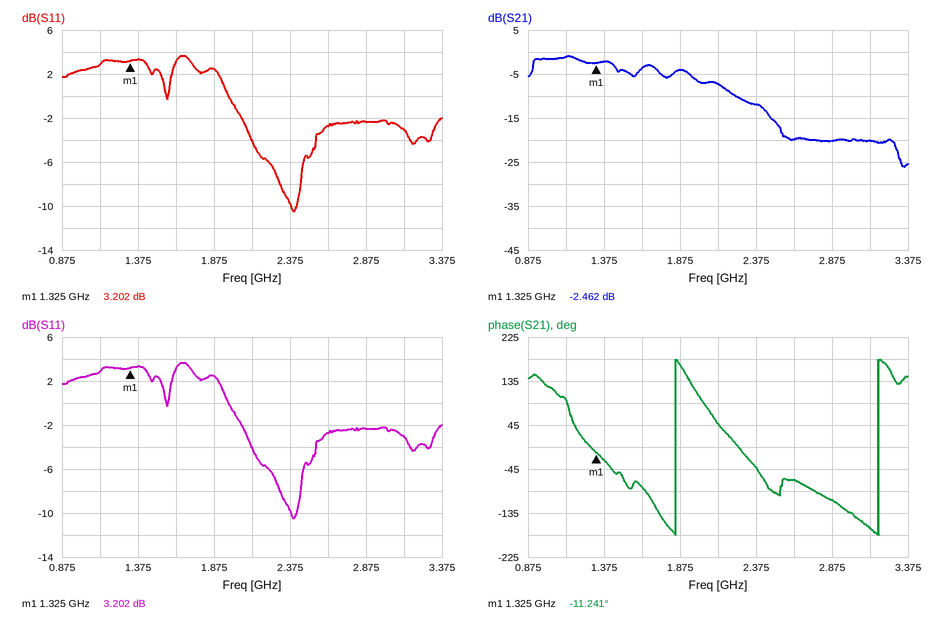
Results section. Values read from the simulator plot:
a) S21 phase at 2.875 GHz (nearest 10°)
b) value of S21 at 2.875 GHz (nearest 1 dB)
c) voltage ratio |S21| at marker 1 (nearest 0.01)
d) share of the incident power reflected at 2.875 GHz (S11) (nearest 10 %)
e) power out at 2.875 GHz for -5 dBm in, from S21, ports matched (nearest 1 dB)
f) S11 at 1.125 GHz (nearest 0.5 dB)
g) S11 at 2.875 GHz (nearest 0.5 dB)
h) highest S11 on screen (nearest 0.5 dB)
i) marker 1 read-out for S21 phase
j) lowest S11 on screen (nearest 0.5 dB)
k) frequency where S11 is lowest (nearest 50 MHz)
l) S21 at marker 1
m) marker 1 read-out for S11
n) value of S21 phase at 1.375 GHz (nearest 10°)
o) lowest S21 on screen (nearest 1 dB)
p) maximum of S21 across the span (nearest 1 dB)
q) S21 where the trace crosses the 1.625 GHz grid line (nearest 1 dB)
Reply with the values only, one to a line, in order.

-110°
-20 dB
0.75
60 %
-25 dBm
3.0 dB
-2.5 dB
3.5 dB
-11.241°
-10.5 dB
2.40 GHz
-2.462 dB
3.202 dB
-30°
-26 dB
-1 dB
-4 dB
